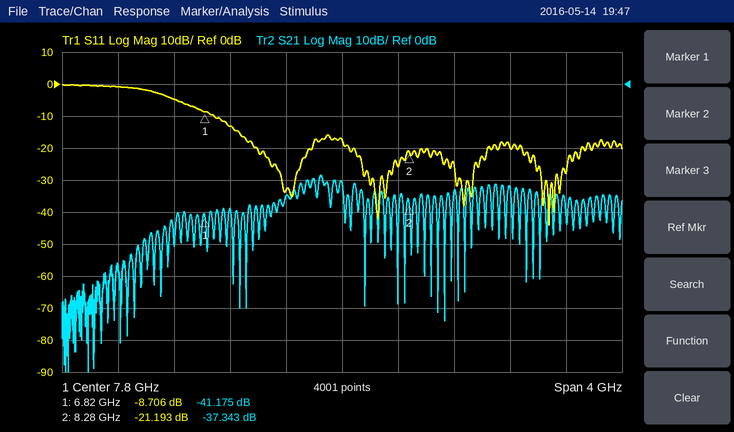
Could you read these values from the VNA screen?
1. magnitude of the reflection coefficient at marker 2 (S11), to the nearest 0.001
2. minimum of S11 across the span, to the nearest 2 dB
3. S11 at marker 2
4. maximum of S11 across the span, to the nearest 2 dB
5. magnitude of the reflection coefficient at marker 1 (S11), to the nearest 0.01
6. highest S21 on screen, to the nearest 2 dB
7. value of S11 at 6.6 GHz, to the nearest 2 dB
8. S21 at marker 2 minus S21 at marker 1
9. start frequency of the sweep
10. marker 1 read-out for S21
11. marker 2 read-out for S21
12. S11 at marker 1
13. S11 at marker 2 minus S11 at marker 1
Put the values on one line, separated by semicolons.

0.087; -44 dB; -21.193 dB; 0 dB; 0.37; -28 dB; -4 dB; 3.832 dB; 5.8 GHz; -41.175 dB; -37.343 dB; -8.706 dB; -12.487 dB
